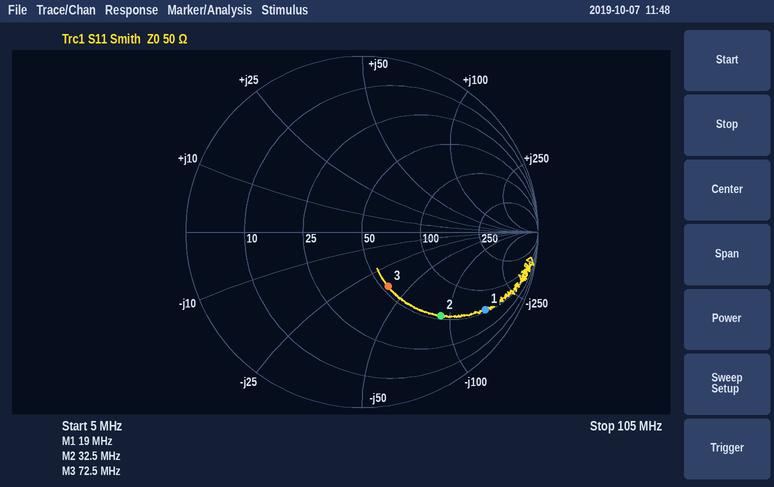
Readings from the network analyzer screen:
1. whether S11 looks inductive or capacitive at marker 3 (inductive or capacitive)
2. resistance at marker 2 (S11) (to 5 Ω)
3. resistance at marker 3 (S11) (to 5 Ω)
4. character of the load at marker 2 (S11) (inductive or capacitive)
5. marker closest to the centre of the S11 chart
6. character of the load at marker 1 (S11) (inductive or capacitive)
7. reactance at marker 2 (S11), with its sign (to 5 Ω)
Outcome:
capacitive
55 Ω
55 Ω
capacitive
marker 3
capacitive
-90 Ω
